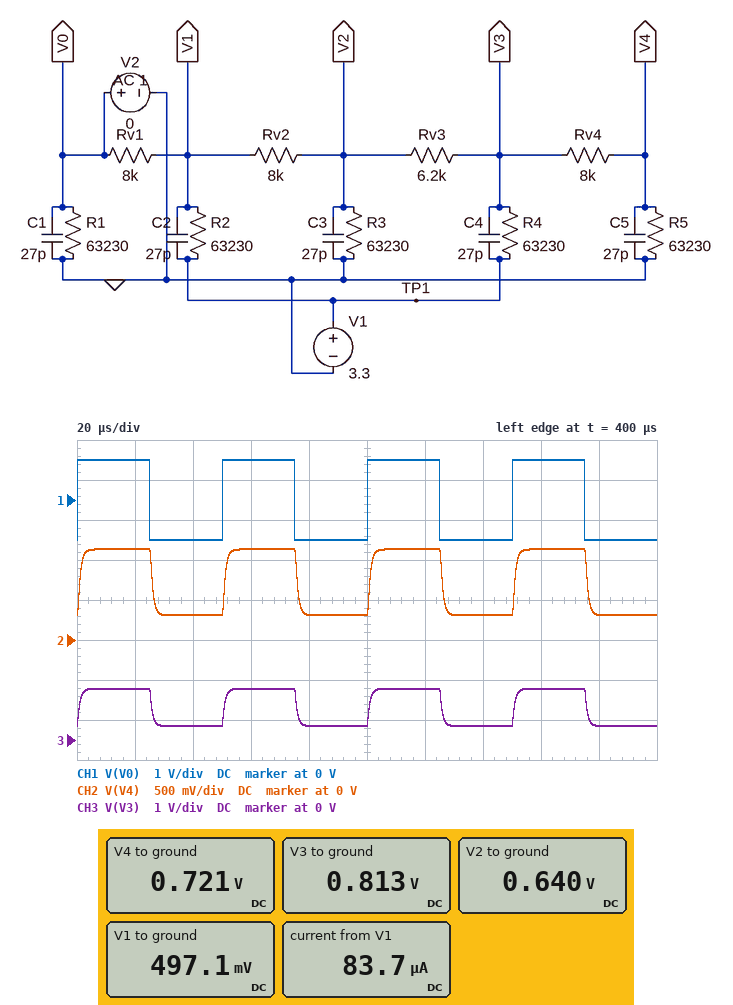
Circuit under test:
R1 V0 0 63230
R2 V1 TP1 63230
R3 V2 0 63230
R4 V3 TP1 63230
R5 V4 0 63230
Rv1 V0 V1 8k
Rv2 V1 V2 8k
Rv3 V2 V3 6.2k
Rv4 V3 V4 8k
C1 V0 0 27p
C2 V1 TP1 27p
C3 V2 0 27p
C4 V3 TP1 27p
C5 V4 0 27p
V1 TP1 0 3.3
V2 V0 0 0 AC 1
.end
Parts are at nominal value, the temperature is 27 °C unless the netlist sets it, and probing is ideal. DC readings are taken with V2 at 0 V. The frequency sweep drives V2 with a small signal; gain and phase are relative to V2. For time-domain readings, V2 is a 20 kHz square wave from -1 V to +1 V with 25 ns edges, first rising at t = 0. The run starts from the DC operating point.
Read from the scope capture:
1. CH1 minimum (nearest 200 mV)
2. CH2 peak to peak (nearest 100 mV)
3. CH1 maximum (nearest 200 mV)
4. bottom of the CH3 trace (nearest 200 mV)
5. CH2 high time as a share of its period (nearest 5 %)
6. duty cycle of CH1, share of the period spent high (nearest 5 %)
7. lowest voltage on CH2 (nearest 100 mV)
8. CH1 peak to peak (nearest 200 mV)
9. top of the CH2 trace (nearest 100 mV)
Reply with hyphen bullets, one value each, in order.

- -1.0 V
- 800 mV
- 1.0 V
- 400 mV
- 50 %
- 50 %
- 300 mV
- 2.0 V
- 1.1 V
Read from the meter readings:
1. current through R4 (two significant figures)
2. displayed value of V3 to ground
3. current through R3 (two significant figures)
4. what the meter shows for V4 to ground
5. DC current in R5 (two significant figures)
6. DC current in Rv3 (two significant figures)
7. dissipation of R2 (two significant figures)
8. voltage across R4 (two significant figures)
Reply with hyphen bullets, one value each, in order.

- 39 µA
- 0.813 V
- 10 µA
- 0.721 V
- 11 µA
- 28 µA
- 120 µW
- 2.5 V
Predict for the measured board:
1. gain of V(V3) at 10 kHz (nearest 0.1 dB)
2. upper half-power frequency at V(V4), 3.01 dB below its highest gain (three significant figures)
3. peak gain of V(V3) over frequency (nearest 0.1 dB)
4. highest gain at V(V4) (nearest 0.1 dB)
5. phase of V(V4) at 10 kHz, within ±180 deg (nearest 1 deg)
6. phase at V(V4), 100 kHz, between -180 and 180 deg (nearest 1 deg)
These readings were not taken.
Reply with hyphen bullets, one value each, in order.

- -6.7 dB
- 176 kHz
- -6.7 dB
- -7.7 dB
- -4 deg
- -40 deg
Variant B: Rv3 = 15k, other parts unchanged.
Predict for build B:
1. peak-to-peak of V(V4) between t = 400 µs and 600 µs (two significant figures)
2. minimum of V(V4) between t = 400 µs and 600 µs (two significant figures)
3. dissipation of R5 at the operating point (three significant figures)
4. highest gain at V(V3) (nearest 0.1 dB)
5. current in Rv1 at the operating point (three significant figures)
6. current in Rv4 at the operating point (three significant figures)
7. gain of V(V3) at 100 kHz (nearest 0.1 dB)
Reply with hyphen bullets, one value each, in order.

- 700 mV
- 490 mV
- 11.2 µW
- -8.1 dB
- 59.2 µA
- 13.3 µA
- -9.4 dB
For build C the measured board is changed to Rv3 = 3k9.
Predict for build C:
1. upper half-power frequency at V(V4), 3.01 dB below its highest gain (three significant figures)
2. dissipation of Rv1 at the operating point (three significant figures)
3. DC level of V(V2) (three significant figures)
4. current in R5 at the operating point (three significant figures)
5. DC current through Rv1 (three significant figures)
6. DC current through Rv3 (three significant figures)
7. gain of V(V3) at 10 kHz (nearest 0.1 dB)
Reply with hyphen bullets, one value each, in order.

- 182 kHz
- 31.8 µW
- 655 mV
- 10.8 µA
- 63.1 µA
- 29.2 µA
- -6.3 dB
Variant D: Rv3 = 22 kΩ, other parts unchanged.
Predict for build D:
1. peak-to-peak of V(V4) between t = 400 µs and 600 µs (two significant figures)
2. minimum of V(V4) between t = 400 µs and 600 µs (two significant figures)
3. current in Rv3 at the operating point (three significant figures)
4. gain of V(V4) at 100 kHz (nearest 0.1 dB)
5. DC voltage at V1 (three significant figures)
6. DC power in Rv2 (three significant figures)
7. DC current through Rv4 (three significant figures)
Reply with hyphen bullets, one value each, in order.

- 630 mV
- 600 mV
- 21.4 µA
- -11.6 dB
- 460 mV
- 1.26 µW
- 14.5 µA
